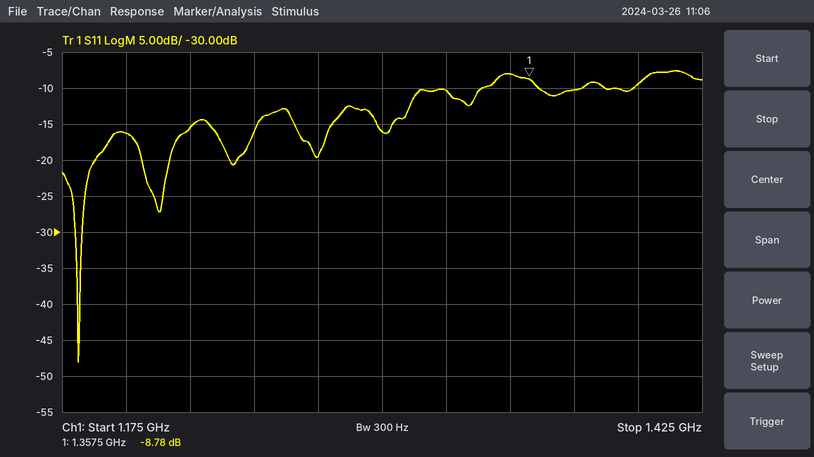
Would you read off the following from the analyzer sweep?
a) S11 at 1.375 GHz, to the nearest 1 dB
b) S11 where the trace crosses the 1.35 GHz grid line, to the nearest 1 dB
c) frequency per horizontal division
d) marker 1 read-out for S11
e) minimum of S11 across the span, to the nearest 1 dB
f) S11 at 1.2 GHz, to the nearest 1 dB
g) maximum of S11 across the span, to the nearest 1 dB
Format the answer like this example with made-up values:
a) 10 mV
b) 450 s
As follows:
a) -10 dB
b) -8 dB
c) 25 MHz
d) -8.78 dB
e) -48 dB
f) -16 dB
g) -8 dB
